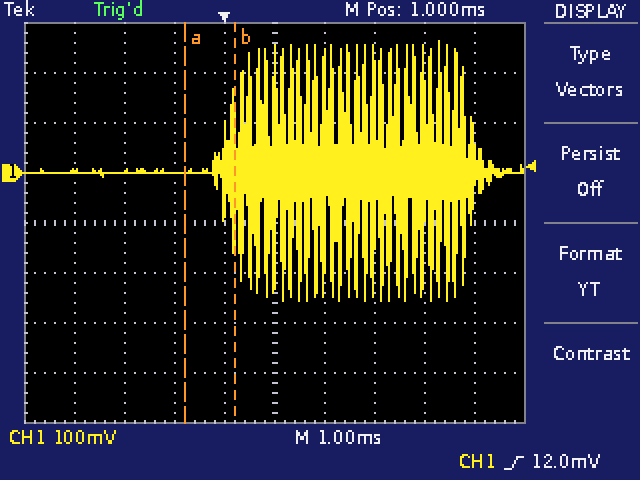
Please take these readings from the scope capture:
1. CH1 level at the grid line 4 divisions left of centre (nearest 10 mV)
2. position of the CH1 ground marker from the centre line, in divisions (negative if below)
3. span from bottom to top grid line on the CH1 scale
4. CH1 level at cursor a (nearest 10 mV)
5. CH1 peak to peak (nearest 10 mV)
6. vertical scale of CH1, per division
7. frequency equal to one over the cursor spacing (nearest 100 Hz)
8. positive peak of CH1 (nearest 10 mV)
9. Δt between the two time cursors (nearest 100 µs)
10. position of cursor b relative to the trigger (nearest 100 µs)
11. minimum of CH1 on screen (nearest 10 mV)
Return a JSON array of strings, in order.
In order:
["0 mV", "+1.0 div", "800 mV", "0 mV", "520 mV", "100 mV", "1.0 kHz", "260 mV", "1.0 ms", "+200 µs", "-260 mV"]
